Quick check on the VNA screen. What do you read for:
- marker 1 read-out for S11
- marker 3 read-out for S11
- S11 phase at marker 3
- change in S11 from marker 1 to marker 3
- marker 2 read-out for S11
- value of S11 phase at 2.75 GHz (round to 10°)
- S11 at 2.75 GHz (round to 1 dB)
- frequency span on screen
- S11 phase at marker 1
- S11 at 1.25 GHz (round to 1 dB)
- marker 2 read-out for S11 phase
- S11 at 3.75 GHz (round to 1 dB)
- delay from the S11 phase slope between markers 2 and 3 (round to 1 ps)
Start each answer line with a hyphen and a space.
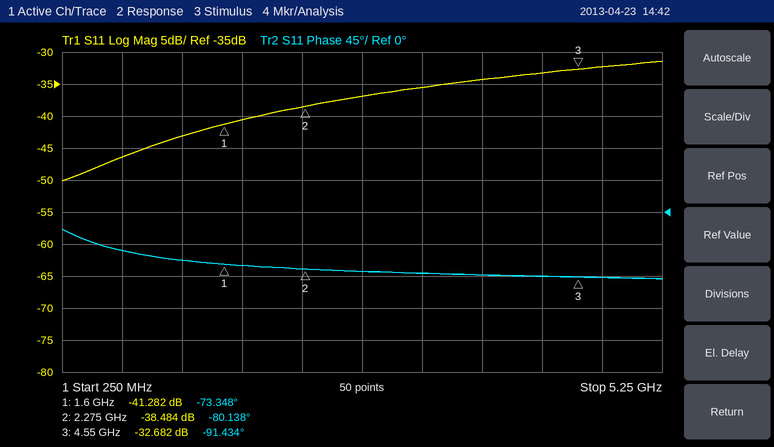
- -41.282 dB
- -32.682 dB
- -91.434°
- 8.600 dB
- -38.484 dB
- -80°
- -37 dB
- 5 GHz
- -73.348°
- -43 dB
- -80.138°
- -34 dB
- 14 ps
